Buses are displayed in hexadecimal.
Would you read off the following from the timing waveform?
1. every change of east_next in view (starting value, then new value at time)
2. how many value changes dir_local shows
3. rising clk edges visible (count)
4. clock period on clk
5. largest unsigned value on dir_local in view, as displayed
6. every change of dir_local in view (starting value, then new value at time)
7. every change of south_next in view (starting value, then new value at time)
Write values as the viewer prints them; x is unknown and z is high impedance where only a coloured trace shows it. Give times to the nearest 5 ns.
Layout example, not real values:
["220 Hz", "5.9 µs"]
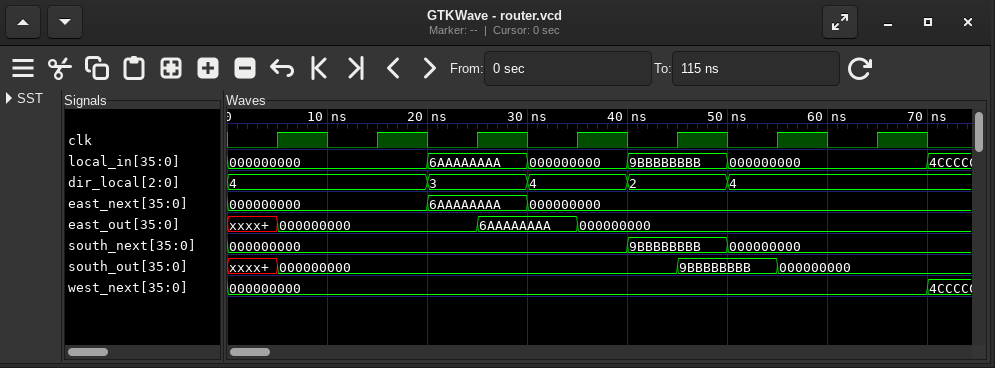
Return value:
["000000000, 6AAAAAAAA at 20 ns, 000000000 at 30 ns", "4", "7", "10 ns", "4", "4, 3 at 20 ns, 4 at 30 ns, 2 at 40 ns, 4 at 50 ns", "000000000, 9BBBBBBBB at 40 ns, 000000000 at 50 ns"]
